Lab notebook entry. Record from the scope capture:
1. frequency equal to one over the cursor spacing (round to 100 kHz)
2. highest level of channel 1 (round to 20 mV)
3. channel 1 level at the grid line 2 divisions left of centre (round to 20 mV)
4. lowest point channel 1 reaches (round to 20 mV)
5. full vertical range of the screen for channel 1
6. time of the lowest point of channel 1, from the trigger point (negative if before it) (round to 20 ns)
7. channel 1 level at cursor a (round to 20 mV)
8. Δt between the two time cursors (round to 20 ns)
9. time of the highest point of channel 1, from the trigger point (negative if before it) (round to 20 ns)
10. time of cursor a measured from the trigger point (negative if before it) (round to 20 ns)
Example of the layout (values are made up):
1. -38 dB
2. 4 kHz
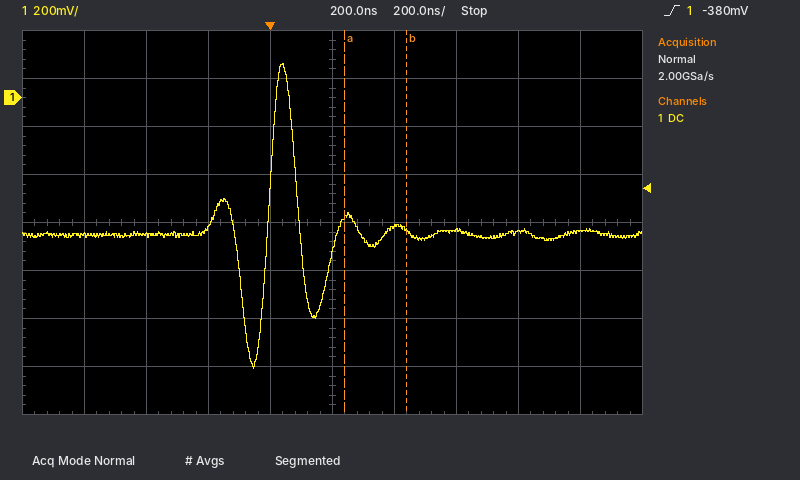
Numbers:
1. 5.0 MHz
2. 140 mV
3. -540 mV
4. -1.12 V
5. 1.6 V
6. -60 ns
7. -500 mV
8. 200 ns
9. +40 ns
10. +240 ns
